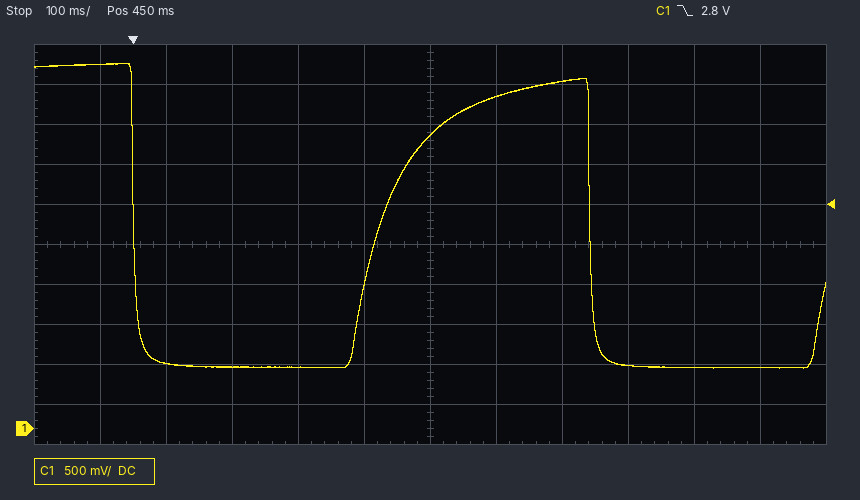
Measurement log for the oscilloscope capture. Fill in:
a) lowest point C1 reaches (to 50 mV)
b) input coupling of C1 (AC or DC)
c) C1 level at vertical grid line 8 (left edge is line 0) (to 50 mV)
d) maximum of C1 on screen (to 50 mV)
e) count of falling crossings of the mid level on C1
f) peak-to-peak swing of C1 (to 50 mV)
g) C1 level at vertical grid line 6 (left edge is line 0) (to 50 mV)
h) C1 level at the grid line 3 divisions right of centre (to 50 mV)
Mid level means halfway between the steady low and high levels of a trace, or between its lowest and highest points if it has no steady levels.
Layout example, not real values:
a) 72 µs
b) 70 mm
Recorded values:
a) 750 mV
b) DC
c) 4.35 V
d) 4.55 V
e) 2
f) 3.80 V
g) 3.65 V
h) 800 mV
